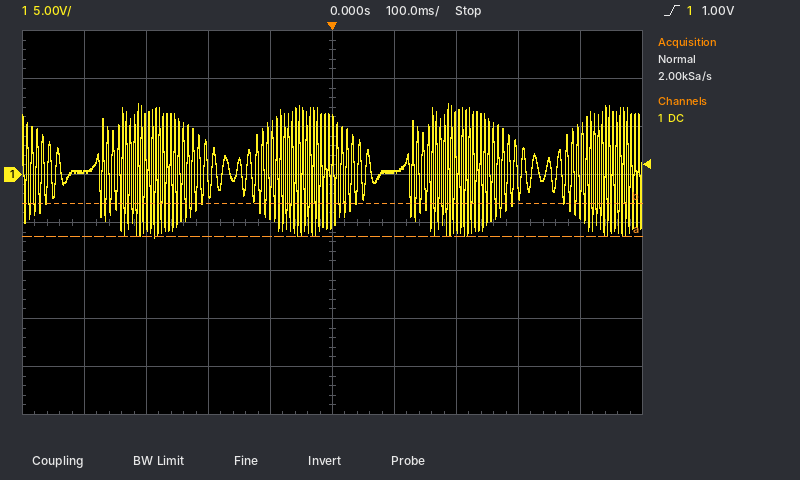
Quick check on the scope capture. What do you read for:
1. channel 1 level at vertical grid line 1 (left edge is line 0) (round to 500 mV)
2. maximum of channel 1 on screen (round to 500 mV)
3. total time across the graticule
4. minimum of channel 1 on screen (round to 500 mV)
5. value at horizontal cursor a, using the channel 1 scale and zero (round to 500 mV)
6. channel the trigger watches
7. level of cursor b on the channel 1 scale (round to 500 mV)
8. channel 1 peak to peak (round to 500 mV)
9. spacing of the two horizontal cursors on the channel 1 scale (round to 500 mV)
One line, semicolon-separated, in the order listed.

500 mV; 7.5 V; 1 s; -6.5 V; -6.5 V; channel 1; -3.0 V; 14.0 V; 3.5 V
